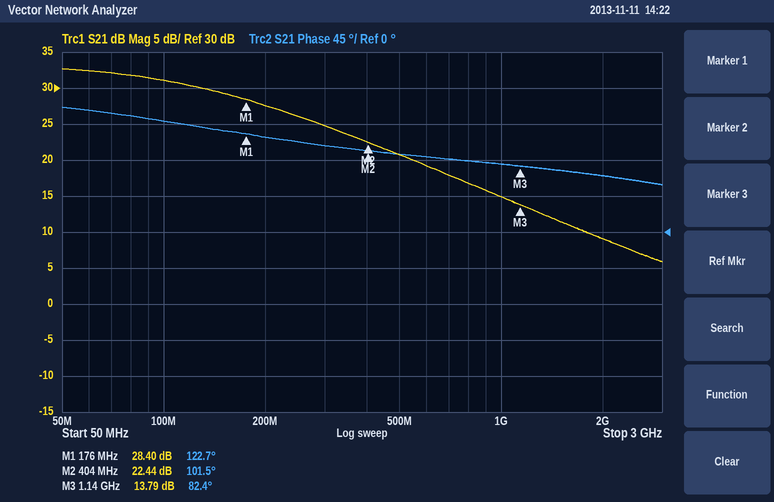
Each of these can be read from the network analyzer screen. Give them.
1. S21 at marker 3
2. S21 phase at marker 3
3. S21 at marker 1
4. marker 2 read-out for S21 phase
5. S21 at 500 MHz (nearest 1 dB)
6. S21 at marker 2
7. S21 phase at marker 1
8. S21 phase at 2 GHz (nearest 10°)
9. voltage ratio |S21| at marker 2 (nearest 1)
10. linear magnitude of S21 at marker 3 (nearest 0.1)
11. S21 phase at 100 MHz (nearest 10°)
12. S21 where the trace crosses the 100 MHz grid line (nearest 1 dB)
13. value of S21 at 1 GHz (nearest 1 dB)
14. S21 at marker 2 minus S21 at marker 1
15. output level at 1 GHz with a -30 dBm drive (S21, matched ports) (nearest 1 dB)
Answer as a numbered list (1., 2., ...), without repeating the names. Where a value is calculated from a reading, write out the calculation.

1. 13.79 dB
2. 82.4°
3. 28.40 dB
4. 101.5°
5. 21 dB
6. 22.44 dB
7. 122.7°
8. 70°
9. 10^(22.44/20) ≈ 13
10. 10^(13.79/20) ≈ 4.9
11. 140°
12. 31 dB
13. 15 dB
14. 22.44 − (28.4) = -5.96 dB
15. -30 dBm + (15 dB) = -15 dBm
